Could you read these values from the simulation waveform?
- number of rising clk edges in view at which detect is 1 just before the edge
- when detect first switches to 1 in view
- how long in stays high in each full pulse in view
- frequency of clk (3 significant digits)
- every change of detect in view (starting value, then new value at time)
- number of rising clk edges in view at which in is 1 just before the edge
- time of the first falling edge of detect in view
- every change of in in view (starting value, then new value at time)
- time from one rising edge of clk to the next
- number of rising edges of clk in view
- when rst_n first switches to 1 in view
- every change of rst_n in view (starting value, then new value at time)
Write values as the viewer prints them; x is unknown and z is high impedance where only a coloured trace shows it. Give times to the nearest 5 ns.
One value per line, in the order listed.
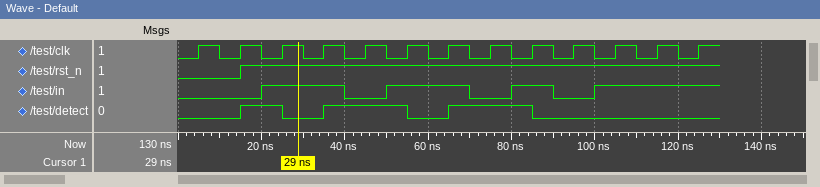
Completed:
5
15 ns
20 ns, 20 ns, 10 ns
100 MHz
0, 1 at 15 ns, 0 at 25 ns, 1 at 35 ns, 0 at 55 ns, 1 at 65 ns, 0 at 85 ns
8
25 ns
0, 1 at 20 ns, 0 at 40 ns, 1 at 50 ns, 0 at 70 ns, 1 at 80 ns, 0 at 90 ns, 1 at 100 ns
10 ns
13
15 ns
0, 1 at 15 ns
